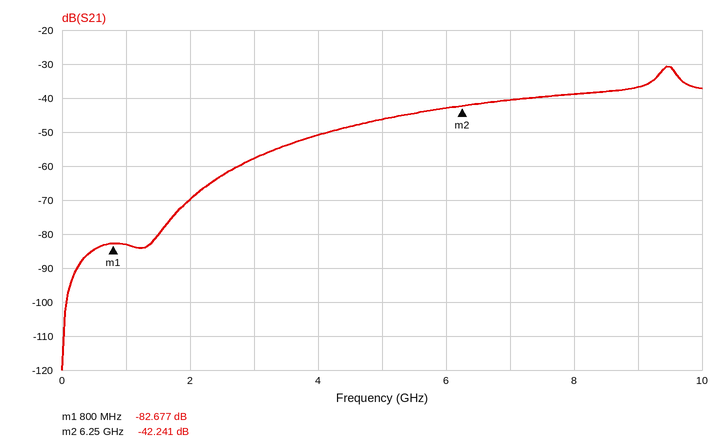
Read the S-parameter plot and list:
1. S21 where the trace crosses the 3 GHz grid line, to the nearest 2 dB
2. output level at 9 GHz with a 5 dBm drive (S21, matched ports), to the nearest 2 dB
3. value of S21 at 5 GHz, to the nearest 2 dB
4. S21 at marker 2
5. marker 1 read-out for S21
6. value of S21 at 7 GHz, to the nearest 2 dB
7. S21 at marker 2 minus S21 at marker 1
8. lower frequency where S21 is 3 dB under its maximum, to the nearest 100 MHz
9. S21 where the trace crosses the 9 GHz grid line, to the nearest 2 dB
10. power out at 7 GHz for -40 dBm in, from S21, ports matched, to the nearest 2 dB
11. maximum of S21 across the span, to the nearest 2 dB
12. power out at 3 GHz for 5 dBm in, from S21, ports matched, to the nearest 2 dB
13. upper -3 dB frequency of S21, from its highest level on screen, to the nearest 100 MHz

-58 dB
-32 dBm
-46 dB
-42.241 dB
-82.677 dB
-40 dB
40.436 dB
9.3 GHz
-36 dB
-80 dBm
-30 dB
-52 dBm
9.6 GHz
